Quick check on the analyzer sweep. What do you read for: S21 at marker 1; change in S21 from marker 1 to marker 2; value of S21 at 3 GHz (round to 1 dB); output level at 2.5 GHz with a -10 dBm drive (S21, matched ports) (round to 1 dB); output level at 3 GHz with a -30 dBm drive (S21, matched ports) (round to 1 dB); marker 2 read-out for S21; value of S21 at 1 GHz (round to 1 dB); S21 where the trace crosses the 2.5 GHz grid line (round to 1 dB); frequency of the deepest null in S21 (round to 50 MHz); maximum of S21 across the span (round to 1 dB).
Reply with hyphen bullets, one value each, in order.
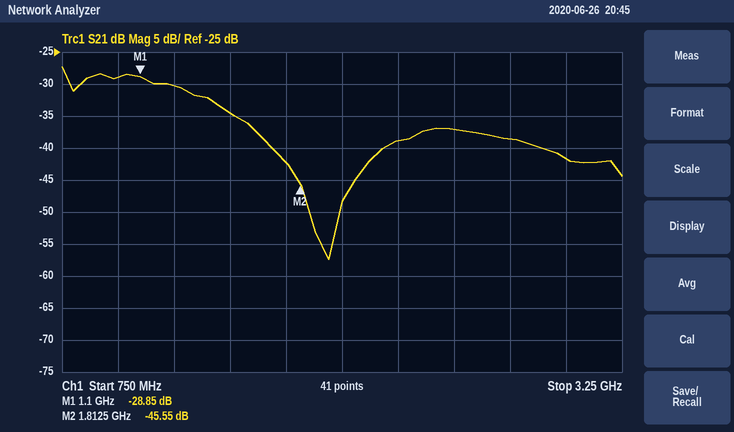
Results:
- -28.85 dB
- -16.70 dB
- -42 dB
- -47 dBm
- -72 dBm
- -45.55 dB
- -29 dB
- -37 dB
- 1.95 GHz
- -27 dB
